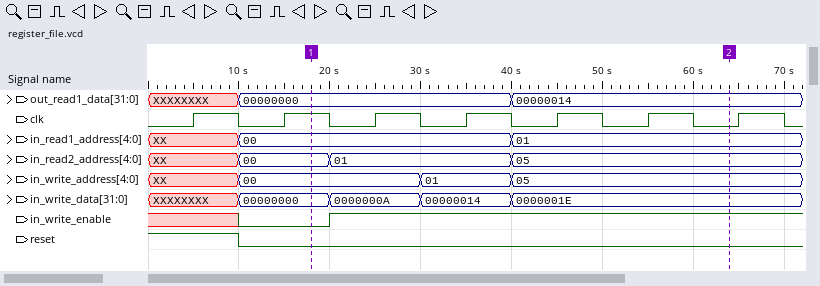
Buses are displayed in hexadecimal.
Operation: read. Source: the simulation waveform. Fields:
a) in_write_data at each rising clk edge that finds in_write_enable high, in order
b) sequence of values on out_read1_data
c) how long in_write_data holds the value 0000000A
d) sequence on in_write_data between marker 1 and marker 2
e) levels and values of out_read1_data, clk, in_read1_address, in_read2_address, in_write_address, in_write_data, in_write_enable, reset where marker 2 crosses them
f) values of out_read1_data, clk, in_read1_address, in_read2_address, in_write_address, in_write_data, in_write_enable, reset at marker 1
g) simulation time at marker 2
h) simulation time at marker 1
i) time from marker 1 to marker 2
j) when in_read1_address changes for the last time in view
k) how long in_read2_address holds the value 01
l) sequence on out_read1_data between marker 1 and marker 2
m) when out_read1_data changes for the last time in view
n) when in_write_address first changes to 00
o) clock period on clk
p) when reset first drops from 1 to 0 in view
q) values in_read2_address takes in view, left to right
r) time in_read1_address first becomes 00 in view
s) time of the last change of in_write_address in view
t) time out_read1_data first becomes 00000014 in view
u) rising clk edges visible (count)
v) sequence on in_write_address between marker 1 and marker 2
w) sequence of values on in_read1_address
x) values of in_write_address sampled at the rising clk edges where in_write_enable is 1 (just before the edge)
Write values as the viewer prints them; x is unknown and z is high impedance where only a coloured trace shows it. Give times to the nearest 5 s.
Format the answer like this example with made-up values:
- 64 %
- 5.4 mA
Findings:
- 0000000A, 00000014, 0000001E, 0000001E, 0000001E
- XXXXXXXX, 00000000, 00000014
- 10 s
- 00000000, 0000000A, 00000014, 0000001E
- out_read1_data=00000014, clk=0, in_read1_address=01, in_read2_address=05, in_write_address=05, in_write_data=0000001E, in_write_enable=1, reset=0
- out_read1_data=00000000, clk=1, in_read1_address=00, in_read2_address=00, in_write_address=00, in_write_data=00000000, in_write_enable=0, reset=0
- 65 s
- 20 s
- 45 s
- 40 s
- 20 s
- 00000000, 00000014
- 40 s
- 10 s
- 10 s
- 10 s
- XX, 00, 01, 05
- 10 s
- 40 s
- 40 s
- 7
- 00, 01, 05
- XX, 00, 01
- 00, 01, 05, 05, 05
